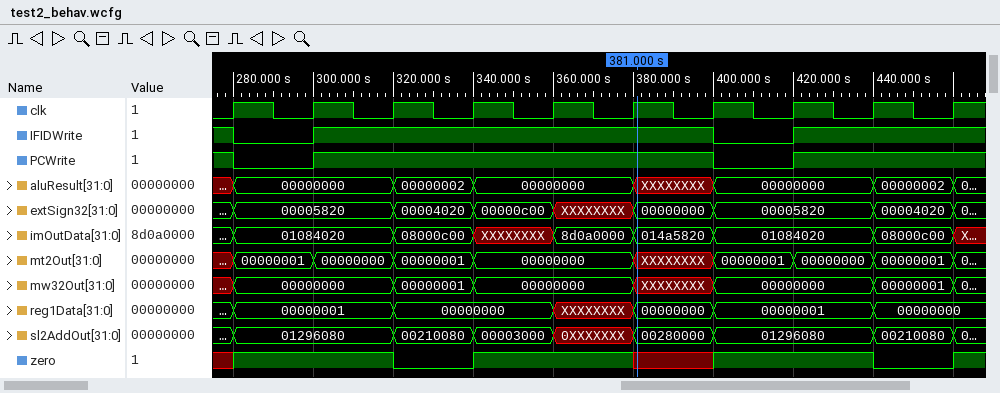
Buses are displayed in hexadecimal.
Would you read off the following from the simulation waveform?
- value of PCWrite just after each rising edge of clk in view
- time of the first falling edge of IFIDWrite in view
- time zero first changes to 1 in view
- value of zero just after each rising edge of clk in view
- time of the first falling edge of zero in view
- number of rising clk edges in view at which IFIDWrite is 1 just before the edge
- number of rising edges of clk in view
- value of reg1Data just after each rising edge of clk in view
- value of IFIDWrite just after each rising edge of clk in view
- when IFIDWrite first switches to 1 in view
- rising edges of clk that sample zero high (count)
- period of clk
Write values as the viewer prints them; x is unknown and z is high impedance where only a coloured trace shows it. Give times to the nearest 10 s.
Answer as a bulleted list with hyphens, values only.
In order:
- 0 1 1 1 1 1 0 1 1 1
- 280 s
- 280 s
- 1 1 0 1 1 x 1 1 0 1
- 320 s
- 8
- 10
- 00000001, 00000001, 00000000, 00000000, XXXXXXXX, 00000000, 00000001, 00000001, 00000000, 00000000
- 0 1 1 1 1 1 0 1 1 1
- 300 s
- 6
- 20 s
